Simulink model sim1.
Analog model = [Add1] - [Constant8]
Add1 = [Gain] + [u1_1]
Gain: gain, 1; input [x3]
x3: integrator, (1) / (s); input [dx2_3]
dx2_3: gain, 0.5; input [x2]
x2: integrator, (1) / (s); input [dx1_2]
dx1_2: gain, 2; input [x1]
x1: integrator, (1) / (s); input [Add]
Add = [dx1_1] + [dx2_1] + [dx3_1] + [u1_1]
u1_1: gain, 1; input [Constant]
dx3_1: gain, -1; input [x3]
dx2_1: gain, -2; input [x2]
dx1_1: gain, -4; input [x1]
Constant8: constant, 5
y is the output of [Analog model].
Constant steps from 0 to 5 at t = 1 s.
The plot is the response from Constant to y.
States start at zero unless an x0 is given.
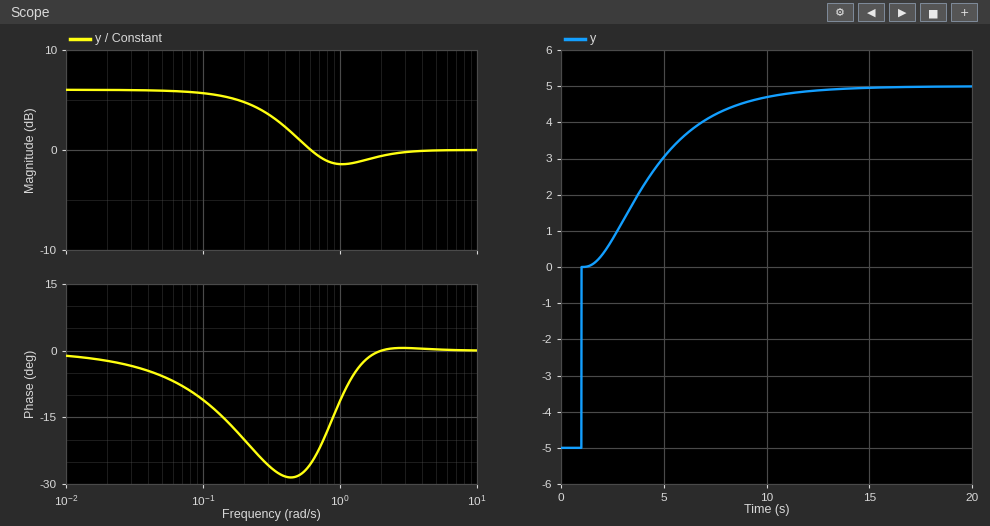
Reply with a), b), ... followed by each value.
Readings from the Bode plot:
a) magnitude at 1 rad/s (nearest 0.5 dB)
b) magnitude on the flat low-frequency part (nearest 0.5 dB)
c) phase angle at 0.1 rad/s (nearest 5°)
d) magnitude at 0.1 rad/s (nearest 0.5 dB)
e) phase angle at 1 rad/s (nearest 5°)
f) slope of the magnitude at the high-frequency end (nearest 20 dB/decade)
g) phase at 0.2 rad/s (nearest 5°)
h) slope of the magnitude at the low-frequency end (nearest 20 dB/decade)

a) -1.5 dB
b) 6.0 dB
c) -10°
d) 5.5 dB
e) -10°
f) 0 dB/decade
g) -20°
h) 0 dB/decade
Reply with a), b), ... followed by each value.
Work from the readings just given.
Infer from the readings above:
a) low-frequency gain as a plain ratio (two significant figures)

a) 2.0
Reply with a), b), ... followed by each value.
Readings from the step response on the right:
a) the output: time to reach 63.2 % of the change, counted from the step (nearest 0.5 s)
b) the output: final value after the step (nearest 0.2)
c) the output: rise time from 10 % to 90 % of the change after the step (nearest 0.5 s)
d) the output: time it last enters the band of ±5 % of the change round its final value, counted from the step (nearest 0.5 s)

a) 2.0 s
b) 5.0
c) 6.0 s
d) 7.5 s
